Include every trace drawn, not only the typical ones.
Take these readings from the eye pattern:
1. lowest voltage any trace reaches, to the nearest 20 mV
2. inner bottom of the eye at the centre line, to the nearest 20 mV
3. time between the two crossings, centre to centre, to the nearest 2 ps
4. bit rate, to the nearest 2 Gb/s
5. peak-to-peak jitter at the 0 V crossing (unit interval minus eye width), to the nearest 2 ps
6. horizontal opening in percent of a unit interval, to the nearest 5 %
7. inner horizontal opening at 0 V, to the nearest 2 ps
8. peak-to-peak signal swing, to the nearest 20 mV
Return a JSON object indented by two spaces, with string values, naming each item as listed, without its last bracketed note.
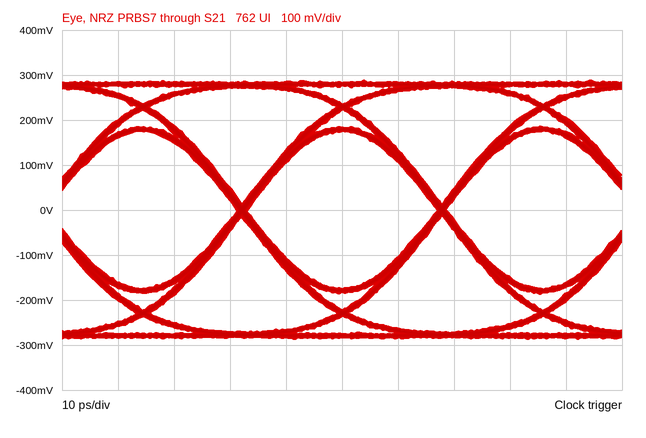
{
  "lowest voltage any trace reaches, to the nearest 20 mV": "-280 mV",
  "inner bottom of the eye at the centre line, to the nearest 20 mV": "-180 mV",
  "time between the two crossings, centre to centre, to the nearest 2 ps": "36 ps",
  "bit rate, to the nearest 2 Gb/s": "28 Gb/s",
  "peak-to-peak jitter at the 0 V crossing (unit interval minus eye width), to the nearest 2 ps": "2 ps",
  "horizontal opening in percent of a unit interval, to the nearest 5 %": "95 %",
  "inner horizontal opening at 0 V, to the nearest 2 ps": "34 ps",
  "peak-to-peak signal swing, to the nearest 20 mV": "580 mV"
}
